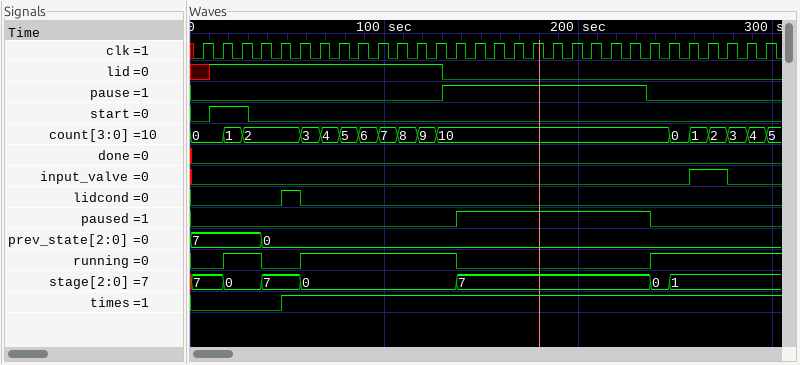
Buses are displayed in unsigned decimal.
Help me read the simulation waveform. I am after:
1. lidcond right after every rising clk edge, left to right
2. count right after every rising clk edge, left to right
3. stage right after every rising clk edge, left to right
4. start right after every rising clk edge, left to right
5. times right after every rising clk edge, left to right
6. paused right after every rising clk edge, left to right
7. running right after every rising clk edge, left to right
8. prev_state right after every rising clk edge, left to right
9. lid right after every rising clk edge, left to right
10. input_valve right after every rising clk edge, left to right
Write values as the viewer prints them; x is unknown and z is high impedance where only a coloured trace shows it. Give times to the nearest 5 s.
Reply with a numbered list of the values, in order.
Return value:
1. 0 0 0 0 1 0 0 0 0 0 0 0 0 0 0 0 0 0 0 0 0 0 0 0 0 0 0 0 0 0
2. 0, 1, 2, 2, 2, 3, 4, 5, 6, 7, 8, 9, 10, 10, 10, 10, 10, 10, 10, 10, 10, 10, 10, 10, 0, 1, 2, 3, 4, 5
3. 7, 0, 0, 7, 7, 0, 0, 0, 0, 0, 0, 0, 0, 7, 7, 7, 7, 7, 7, 7, 7, 7, 7, 0, 1, 1, 1, 1, 1, 1
4. 0 1 1 0 0 0 0 0 0 0 0 0 0 0 0 0 0 0 0 0 0 0 0 0 0 0 0 0 0 0
5. 0 0 0 0 1 1 1 1 1 1 1 1 1 1 1 1 1 1 1 1 1 1 1 1 1 1 1 1 1 1
6. 0 0 0 0 0 0 0 0 0 0 0 0 0 1 1 1 1 1 1 1 1 1 1 0 0 0 0 0 0 0
7. 0 1 1 0 0 1 1 1 1 1 1 1 1 0 0 0 0 0 0 0 0 0 0 1 1 1 1 1 1 1
8. 7, 7, 7, 0, 0, 0, 0, 0, 0, 0, 0, 0, 0, 0, 0, 0, 0, 0, 0, 0, 0, 0, 0, 0, 0, 0, 0, 0, 0, 0
9. x 1 1 1 1 1 1 1 1 1 1 1 1 0 0 0 0 0 0 0 0 0 0 0 0 0 0 0 0 0
10. 0 0 0 0 0 0 0 0 0 0 0 0 0 0 0 0 0 0 0 0 0 0 0 0 0 1 1 0 0 0
